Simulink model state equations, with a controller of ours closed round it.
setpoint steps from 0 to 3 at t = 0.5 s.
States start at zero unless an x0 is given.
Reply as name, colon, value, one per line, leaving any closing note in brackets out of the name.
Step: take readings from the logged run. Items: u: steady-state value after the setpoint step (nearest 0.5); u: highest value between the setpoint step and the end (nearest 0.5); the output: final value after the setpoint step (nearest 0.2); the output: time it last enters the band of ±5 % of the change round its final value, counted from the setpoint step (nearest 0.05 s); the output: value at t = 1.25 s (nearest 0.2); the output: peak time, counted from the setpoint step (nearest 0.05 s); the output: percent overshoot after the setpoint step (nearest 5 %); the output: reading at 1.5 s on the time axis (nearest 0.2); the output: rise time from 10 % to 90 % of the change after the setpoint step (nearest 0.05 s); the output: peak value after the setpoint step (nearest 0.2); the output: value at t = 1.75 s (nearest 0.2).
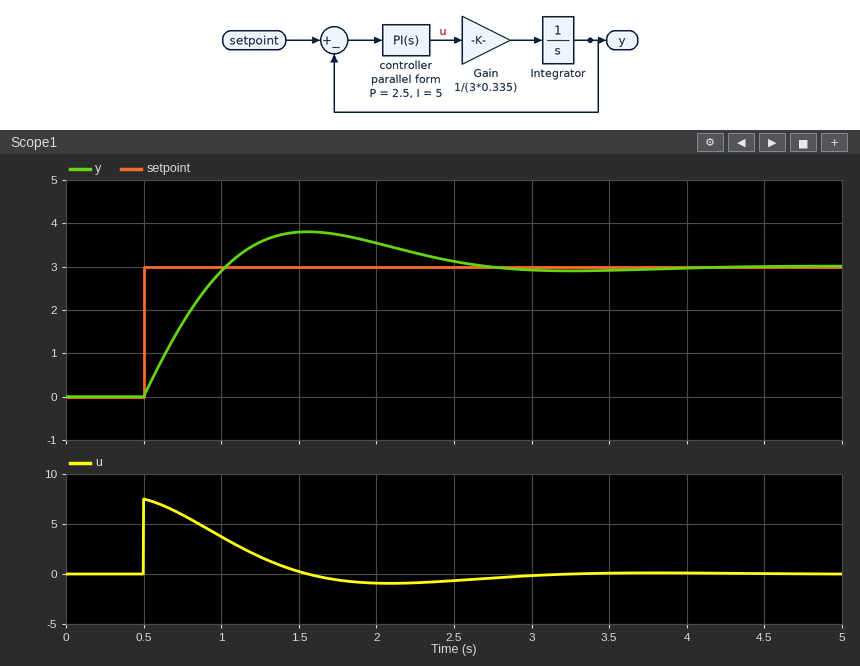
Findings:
u: steady-state value after the setpoint step: 0.0
u: highest value between the setpoint step and the end: 7.5
the output: final value after the setpoint step: 3.0
the output: time it last enters the band of ±5 % of the change round its final value, counted from the setpoint step: 1.95 s
the output: value at t = 1.25 s: 3.6
the output: peak time, counted from the setpoint step: 1.05 s
the output: percent overshoot after the setpoint step: 25 %
the output: reading at 1.5 s on the time axis: 3.8
the output: rise time from 10 % to 90 % of the change after the setpoint step: 0.40 s
the output: peak value after the setpoint step: 3.8
the output: value at t = 1.75 s: 3.8
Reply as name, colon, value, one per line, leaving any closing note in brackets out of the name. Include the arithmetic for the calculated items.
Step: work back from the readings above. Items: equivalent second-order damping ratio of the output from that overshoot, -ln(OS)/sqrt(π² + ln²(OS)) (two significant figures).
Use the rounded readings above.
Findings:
equivalent second-order damping ratio of the output from that overshoot, -ln(OS)/sqrt(π² + ln²(OS)): ln(0.25) = -1.386; 1.386 / sqrt(9.870 + 1.922) = 0.40
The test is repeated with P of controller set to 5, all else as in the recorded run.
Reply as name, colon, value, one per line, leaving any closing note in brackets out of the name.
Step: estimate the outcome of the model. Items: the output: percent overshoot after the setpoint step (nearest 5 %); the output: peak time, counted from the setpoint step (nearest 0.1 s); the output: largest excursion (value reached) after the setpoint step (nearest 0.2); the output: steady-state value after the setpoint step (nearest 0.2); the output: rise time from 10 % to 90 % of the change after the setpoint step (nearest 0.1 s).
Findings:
the output: percent overshoot after the setpoint step: 10 %
the output: peak time, counted from the setpoint step: 0.9 s
the output: largest excursion (value reached) after the setpoint step: 3.4
the output: steady-state value after the setpoint step: 3.0
the output: rise time from 10 % to 90 % of the change after the setpoint step: 0.3 s
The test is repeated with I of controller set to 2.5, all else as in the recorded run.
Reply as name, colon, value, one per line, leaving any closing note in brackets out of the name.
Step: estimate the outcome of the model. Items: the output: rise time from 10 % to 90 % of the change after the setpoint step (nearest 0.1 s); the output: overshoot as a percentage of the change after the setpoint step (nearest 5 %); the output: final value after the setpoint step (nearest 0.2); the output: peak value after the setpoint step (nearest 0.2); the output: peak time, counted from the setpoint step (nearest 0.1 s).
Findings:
the output: rise time from 10 % to 90 % of the change after the setpoint step: 0.5 s
the output: overshoot as a percentage of the change after the setpoint step: 20 %
the output: final value after the setpoint step: 3.0
the output: peak value after the setpoint step: 3.6
the output: peak time, counted from the setpoint step: 1.4 s
